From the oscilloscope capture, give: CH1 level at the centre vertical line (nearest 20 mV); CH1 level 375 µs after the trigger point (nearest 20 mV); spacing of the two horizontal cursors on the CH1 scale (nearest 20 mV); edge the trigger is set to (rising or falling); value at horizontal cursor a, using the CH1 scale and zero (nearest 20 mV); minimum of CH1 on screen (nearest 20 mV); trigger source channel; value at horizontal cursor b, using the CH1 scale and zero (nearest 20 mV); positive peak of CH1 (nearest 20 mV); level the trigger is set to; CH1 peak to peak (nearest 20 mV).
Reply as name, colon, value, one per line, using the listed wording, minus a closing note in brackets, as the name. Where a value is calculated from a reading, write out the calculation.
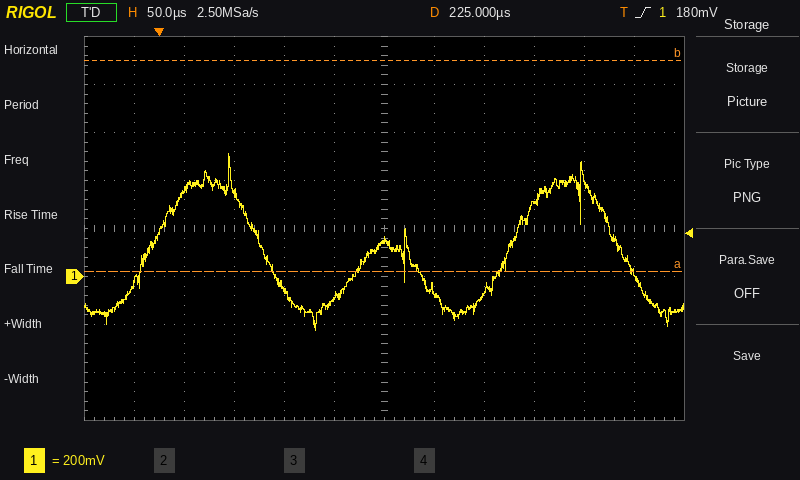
CH1 level at the centre vertical line: 160 mV
CH1 level 375 µs after the trigger point: 300 mV
spacing of the two horizontal cursors on the CH1 scale: 880 mV
edge the trigger is set to: rising
value at horizontal cursor a, using the CH1 scale and zero: 20 mV
minimum of CH1 on screen: -220 mV
trigger source channel: CH1
value at horizontal cursor b, using the CH1 scale and zero: 900 mV
positive peak of CH1: 520 mV
level the trigger is set to: 180 mV
CH1 peak to peak: 520 mV − (-220 mV) = 740 mV
